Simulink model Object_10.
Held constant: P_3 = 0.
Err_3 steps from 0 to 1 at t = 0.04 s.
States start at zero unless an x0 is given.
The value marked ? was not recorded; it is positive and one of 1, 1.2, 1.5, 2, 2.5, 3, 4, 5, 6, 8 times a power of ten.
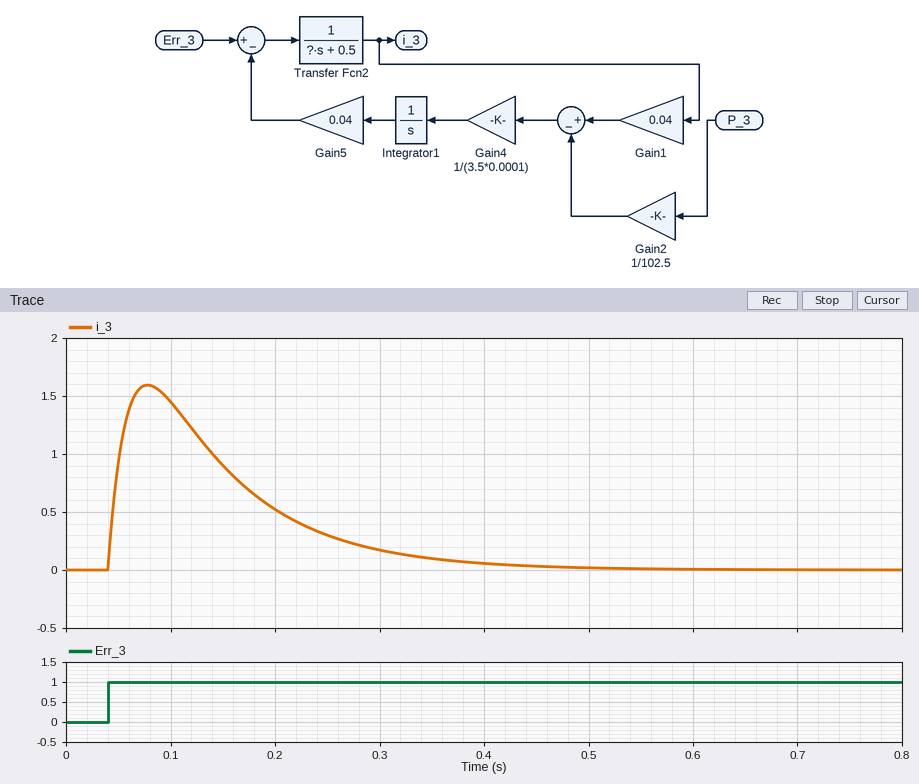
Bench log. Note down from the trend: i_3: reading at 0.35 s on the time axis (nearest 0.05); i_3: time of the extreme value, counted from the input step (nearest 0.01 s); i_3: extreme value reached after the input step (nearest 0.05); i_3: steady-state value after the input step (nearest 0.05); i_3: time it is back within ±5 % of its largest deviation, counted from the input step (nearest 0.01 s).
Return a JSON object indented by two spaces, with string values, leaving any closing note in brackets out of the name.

{
  "i_3: reading at 0.35 s on the time axis": "0.10",
  "i_3: time of the extreme value, counted from the input step": "0.04 s",
  "i_3: extreme value reached after the input step": "1.60",
  "i_3: steady-state value after the input step": "0.00",
  "i_3: time it is back within ±5 % of its largest deviation, counted from the input step": "0.33 s"
}
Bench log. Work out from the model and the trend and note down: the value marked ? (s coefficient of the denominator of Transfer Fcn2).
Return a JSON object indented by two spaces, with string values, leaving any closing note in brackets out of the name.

{
  "the value marked ?": "0.008"
}
